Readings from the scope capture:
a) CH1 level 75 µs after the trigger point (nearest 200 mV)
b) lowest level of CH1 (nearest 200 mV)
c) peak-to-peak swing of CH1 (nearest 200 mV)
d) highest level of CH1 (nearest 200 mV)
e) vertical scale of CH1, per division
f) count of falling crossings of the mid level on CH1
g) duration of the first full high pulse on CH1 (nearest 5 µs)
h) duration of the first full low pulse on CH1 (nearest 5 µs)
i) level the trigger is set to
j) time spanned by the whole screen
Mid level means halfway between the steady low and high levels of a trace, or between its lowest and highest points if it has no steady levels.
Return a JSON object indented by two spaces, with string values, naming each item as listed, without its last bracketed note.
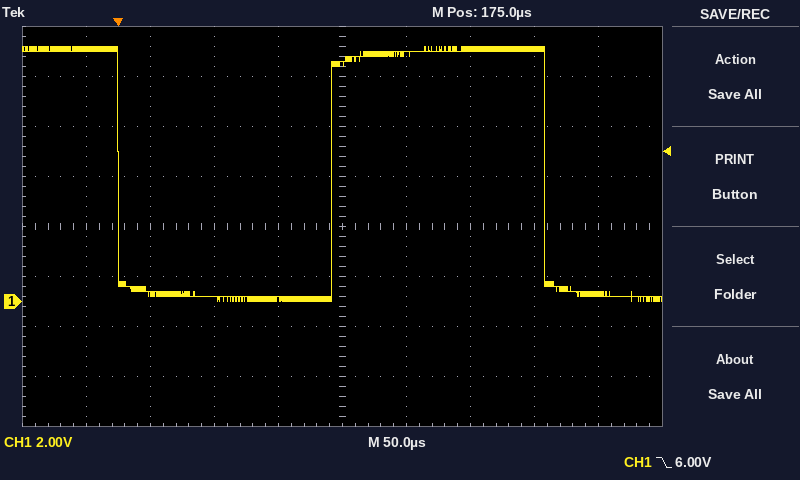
{
  "CH1 level 75 µs after the trigger point": "200 mV",
  "lowest level of CH1": "0.0 V",
  "peak-to-peak swing of CH1": "10.2 V",
  "highest level of CH1": "10.2 V",
  "vertical scale of CH1, per division": "2 V",
  "count of falling crossings of the mid level on CH1": "2",
  "duration of the first full high pulse on CH1": "165 µs",
  "duration of the first full low pulse on CH1": "165 µs",
  "level the trigger is set to": "6.00 V",
  "time spanned by the whole screen": "500 µs"
}
